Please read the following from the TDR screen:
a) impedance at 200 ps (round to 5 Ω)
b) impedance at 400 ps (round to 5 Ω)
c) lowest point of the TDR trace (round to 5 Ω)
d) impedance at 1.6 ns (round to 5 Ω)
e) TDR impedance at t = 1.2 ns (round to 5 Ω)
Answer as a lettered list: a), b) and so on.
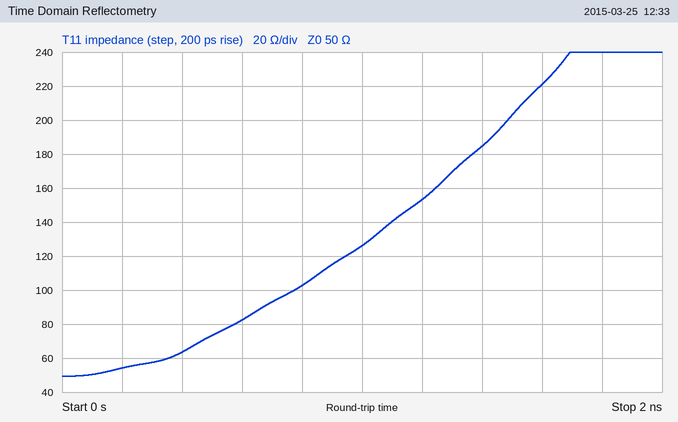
a) 55 Ω
b) 65 Ω
c) 50 Ω
d) 220 Ω
e) 155 Ω
